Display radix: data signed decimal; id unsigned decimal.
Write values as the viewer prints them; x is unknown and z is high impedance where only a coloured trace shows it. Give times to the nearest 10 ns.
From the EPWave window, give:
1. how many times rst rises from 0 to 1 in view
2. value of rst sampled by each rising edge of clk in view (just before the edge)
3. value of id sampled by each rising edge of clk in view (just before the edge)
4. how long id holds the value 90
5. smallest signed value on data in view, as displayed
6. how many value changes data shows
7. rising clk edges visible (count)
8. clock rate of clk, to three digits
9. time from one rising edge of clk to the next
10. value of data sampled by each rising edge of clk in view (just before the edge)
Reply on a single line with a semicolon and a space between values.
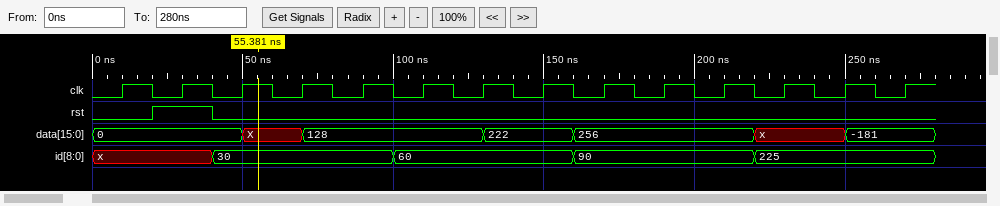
1; 0 1 0 0 0 0 0 0 0 0 0 0 0 0; x, x, 30, 30, 30, 60, 60, 60, 90, 90, 90, 225, 225, 225; 60 ns; -181; 6; 14; 50.0 MHz; 20 ns; 0, 0, 0, X, 128, 128, 128, 222, 256, 256, 256, x, x, -181
